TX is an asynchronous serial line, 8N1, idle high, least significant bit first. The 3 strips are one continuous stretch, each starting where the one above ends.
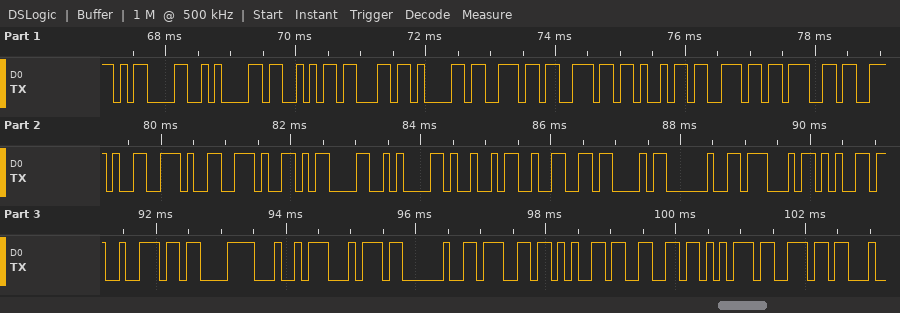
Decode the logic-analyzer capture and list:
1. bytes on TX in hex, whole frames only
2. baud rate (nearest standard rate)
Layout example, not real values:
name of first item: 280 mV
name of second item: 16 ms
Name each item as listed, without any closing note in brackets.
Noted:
bytes on TX in hex, whole frames only: 0D 0A 53 63 61 6E 6E 69 6E 67 2E 2E 2E 0D 0A 49 32 43 20 47 65 72 C3 A4 74 20 67 65 66 75 6E
baud rate: 9600 baud
